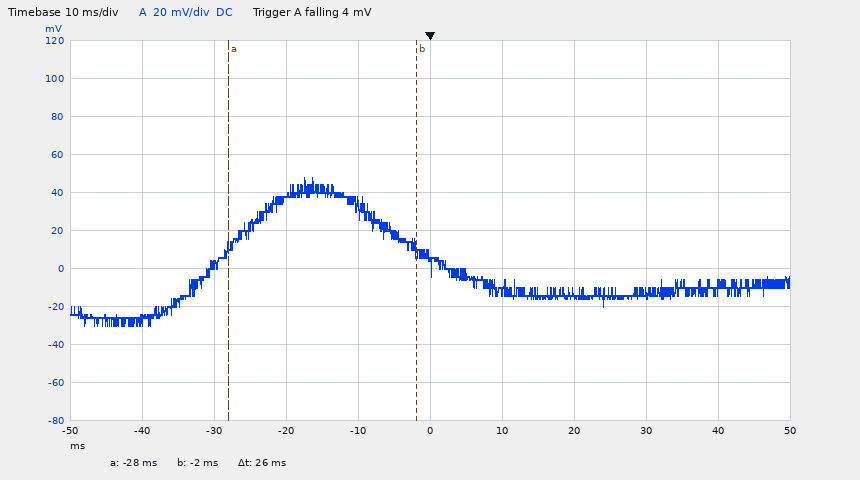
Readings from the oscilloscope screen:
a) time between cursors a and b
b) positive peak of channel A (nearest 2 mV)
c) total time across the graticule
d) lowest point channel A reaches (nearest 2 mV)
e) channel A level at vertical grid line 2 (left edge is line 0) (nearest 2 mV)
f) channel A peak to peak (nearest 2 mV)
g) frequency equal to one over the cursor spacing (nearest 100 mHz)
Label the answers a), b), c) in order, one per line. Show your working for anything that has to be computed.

a) 26 ms
b) 48 mV
c) 100 ms
d) -30 mV
e) 2 mV
f) 48 mV − (-30 mV) = 78 mV
g) 1 / 26 ms ≈ 38.5 Hz
